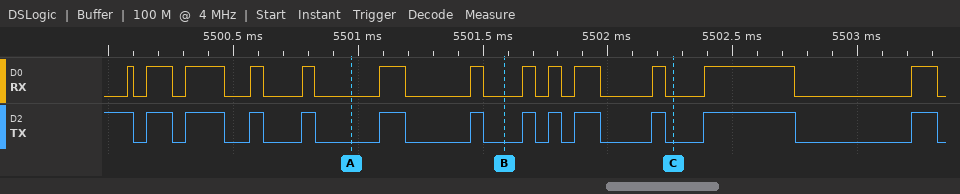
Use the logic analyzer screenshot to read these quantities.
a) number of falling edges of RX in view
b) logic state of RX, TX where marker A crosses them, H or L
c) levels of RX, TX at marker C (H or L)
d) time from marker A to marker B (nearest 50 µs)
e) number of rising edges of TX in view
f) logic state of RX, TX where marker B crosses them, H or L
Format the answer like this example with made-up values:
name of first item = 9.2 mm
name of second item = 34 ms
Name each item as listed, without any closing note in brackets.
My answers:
number of falling edges of RX in view = 13
logic state of RX, TX where marker A crosses them, H or L = RX=L, TX=L
levels of RX, TX at marker C = RX=L, TX=L
time from marker A to marker B = 600 µs
number of rising edges of TX in view = 12
logic state of RX, TX where marker B crosses them, H or L = RX=L, TX=L
